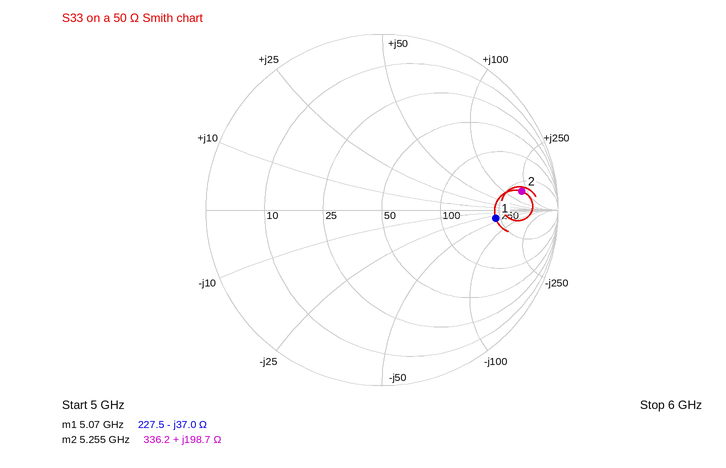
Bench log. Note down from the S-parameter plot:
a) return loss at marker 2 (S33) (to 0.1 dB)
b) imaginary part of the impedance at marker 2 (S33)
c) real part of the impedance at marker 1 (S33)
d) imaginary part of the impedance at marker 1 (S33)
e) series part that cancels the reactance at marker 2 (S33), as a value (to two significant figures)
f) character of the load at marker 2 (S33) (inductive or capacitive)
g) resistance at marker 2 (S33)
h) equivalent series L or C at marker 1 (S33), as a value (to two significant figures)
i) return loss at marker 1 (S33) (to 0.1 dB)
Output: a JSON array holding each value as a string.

["1.9 dB", "+198.7 Ω", "227.5 Ω", "-37.0 Ω", "150 fF", "inductive", "336.2 Ω", "850 fF", "3.8 dB"]
